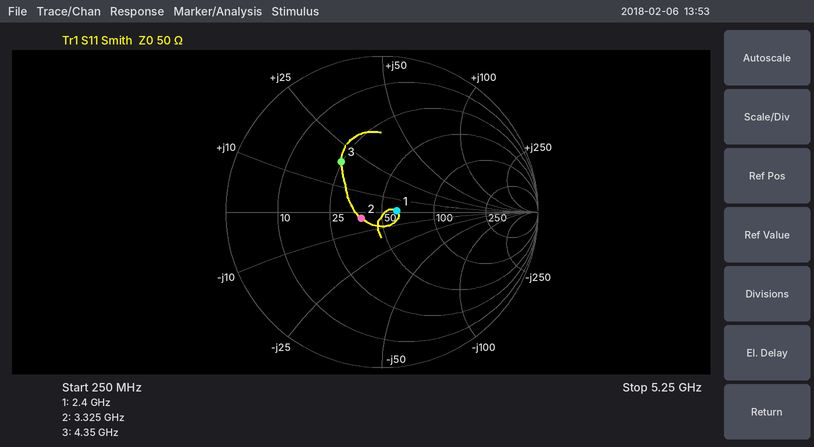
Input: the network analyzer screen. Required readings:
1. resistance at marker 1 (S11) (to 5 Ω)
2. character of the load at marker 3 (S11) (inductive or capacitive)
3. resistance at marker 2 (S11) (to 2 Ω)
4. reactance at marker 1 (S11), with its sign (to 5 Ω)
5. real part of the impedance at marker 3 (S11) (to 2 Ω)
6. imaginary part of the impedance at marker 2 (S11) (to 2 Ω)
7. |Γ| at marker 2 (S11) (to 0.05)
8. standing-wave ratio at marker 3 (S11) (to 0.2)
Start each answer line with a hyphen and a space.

- 60 Ω
- inductive
- 38 Ω
- 0 Ω
- 24 Ω
- -4 Ω
- 0.15
- 2.4
